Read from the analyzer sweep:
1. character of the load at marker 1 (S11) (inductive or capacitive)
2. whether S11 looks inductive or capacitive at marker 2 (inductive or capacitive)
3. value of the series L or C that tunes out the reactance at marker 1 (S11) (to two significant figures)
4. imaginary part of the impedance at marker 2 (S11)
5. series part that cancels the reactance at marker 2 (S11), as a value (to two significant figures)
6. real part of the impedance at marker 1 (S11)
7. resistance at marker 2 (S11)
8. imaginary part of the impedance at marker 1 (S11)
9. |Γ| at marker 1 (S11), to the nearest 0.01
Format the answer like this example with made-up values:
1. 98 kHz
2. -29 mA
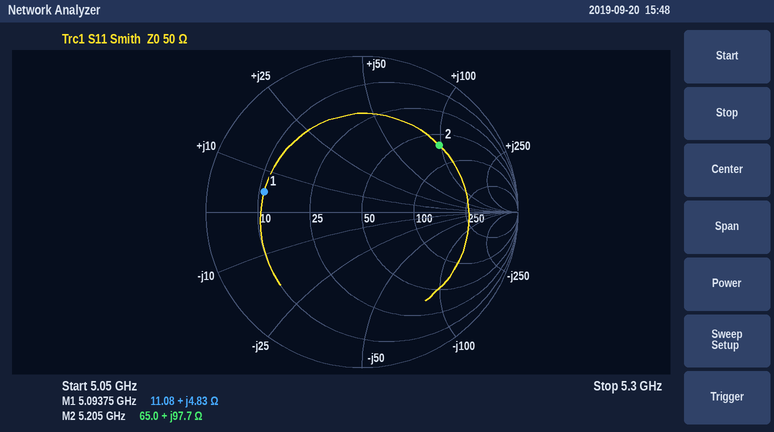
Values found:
1. inductive
2. inductive
3. 6.5 pF
4. +97.7 Ω
5. 310 fF
6. 11.08 Ω
7. 65.0 Ω
8. +4.83 Ω
9. 0.64
